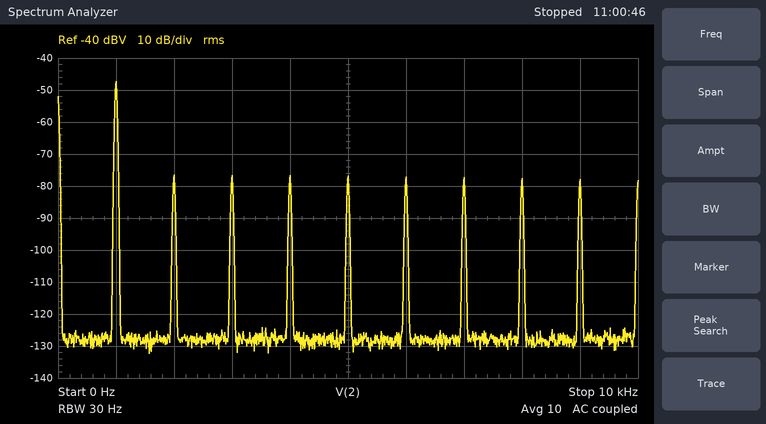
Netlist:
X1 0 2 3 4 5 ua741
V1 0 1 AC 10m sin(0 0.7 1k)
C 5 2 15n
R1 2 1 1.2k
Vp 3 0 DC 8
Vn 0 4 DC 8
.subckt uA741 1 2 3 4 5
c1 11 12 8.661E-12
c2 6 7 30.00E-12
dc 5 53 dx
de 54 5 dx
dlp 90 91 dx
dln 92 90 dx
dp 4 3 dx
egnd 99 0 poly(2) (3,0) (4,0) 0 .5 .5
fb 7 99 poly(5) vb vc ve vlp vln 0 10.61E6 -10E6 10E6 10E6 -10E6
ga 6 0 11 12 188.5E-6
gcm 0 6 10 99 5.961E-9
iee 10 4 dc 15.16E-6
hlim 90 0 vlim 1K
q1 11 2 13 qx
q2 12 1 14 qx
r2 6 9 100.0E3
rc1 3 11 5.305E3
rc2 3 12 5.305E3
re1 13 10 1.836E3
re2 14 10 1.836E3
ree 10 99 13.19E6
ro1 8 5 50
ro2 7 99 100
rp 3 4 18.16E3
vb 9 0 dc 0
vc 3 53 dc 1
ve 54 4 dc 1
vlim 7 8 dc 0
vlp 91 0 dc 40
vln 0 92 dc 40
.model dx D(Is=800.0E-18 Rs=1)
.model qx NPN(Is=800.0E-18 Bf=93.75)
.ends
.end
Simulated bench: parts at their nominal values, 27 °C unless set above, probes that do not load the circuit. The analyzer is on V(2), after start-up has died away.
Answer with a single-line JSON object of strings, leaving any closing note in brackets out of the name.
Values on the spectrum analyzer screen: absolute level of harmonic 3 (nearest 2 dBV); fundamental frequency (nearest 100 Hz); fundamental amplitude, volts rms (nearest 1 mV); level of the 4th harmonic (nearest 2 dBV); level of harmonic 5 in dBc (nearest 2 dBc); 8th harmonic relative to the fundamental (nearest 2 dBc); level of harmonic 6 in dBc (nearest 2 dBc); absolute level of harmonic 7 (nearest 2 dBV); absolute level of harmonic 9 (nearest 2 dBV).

{"absolute level of harmonic 3": "-76 dBV", "fundamental frequency": "1.0 kHz", "fundamental amplitude, volts rms": "4 mV", "level of the 4th harmonic": "-76 dBV", "level of harmonic 5 in dBc": "-30 dBc", "8th harmonic relative to the fundamental": "-30 dBc", "level of harmonic 6 in dBc": "-30 dBc", "absolute level of harmonic 7": "-78 dBV", "absolute level of harmonic 9": "-78 dBV"}
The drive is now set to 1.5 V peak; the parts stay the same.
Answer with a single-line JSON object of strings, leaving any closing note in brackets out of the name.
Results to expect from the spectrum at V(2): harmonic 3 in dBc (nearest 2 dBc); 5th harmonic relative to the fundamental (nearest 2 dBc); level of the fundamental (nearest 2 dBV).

{"harmonic 3 in dBc": "-4 dBc", "5th harmonic relative to the fundamental": "-14 dBc", "level of the fundamental": "-6 dBV"}
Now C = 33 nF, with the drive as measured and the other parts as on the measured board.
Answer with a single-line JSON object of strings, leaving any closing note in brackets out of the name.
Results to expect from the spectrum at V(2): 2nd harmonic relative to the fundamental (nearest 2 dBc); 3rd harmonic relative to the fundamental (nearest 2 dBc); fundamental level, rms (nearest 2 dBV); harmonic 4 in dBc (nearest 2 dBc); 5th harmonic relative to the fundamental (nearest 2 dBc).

{"2nd harmonic relative to the fundamental": "-24 dBc", "3rd harmonic relative to the fundamental": "-24 dBc", "fundamental level, rms": "-54 dBV", "harmonic 4 in dBc": "-24 dBc", "5th harmonic relative to the fundamental": "-24 dBc"}
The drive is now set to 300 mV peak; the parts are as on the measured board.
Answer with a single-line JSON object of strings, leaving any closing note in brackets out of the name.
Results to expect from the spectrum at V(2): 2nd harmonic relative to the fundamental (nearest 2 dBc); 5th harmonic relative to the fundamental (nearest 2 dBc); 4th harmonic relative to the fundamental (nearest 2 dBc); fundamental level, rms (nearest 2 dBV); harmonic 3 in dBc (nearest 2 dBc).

{"2nd harmonic relative to the fundamental": "-24 dBc", "5th harmonic relative to the fundamental": "-24 dBc", "4th harmonic relative to the fundamental": "-24 dBc", "fundamental level, rms": "-54 dBV", "harmonic 3 in dBc": "-24 dBc"}
